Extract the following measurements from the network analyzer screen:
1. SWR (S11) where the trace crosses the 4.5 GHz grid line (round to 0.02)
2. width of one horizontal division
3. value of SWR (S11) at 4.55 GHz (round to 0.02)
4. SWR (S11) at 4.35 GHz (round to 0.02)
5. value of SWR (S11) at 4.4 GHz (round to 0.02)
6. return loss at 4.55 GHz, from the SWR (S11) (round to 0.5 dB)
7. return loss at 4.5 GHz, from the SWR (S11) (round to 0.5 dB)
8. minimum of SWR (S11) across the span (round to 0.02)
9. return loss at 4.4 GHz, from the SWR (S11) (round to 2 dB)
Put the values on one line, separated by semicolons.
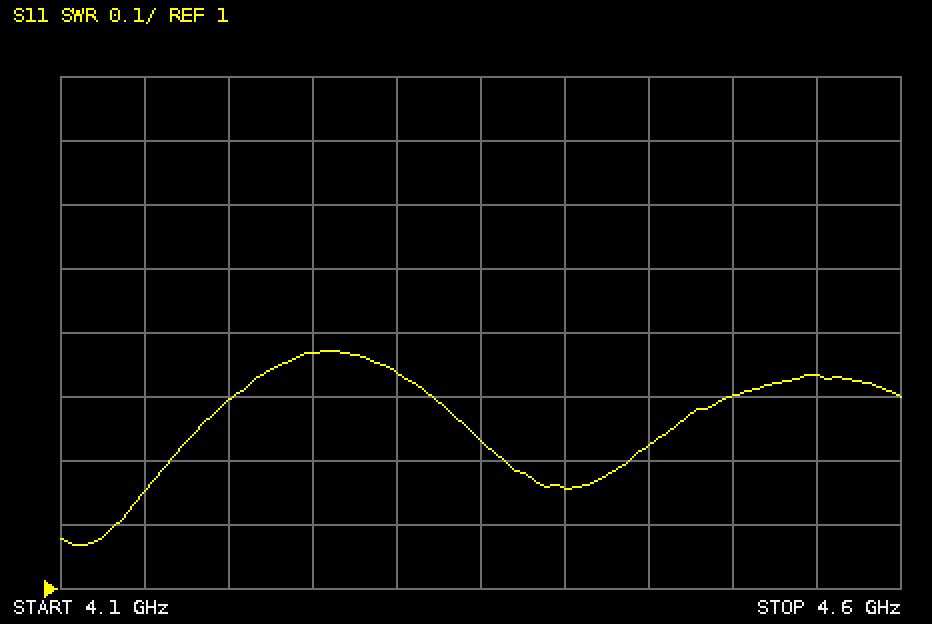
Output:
1.30; 50 MHz; 1.34; 1.24; 1.16; 17.0 dB; 17.5 dB; 1.06; 22 dB
